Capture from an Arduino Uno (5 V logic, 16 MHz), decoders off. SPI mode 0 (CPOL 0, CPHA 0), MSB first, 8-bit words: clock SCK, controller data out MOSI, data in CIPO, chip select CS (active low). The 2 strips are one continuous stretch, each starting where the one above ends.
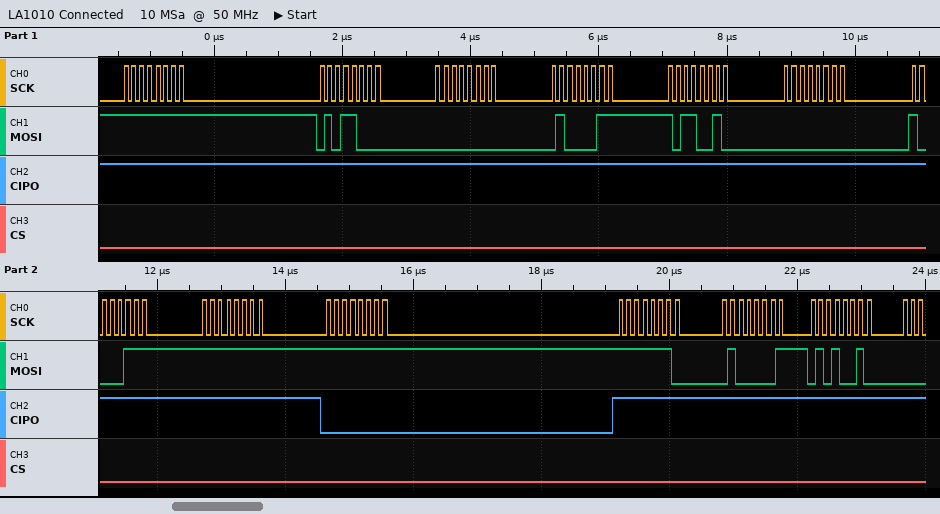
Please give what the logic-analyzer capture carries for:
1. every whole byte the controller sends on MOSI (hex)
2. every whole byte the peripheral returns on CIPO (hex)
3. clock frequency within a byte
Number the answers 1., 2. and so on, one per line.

1. 0xFF 0x58 0x00 0x43 0xB2 0x00 0x87 0xFF 0xFF 0xFE 0x41 0x52
2. 0xFF 0xFF 0xFF 0xFF 0xFF 0xFF 0xFF 0xFF 0x00 0xFF 0xFF 0xFF
3. 8 MHz
